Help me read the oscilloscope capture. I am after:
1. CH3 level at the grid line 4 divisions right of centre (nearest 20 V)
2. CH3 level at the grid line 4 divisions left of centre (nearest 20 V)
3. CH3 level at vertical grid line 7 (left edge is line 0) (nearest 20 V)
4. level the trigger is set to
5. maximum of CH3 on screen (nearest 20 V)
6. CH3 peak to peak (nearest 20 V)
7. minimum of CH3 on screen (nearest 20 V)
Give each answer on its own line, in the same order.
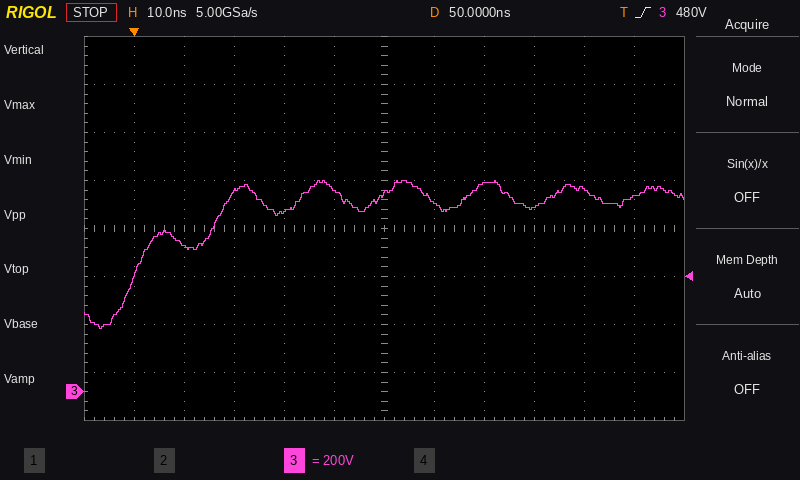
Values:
840 V
600 V
780 V
480 V
880 V
620 V
260 V
